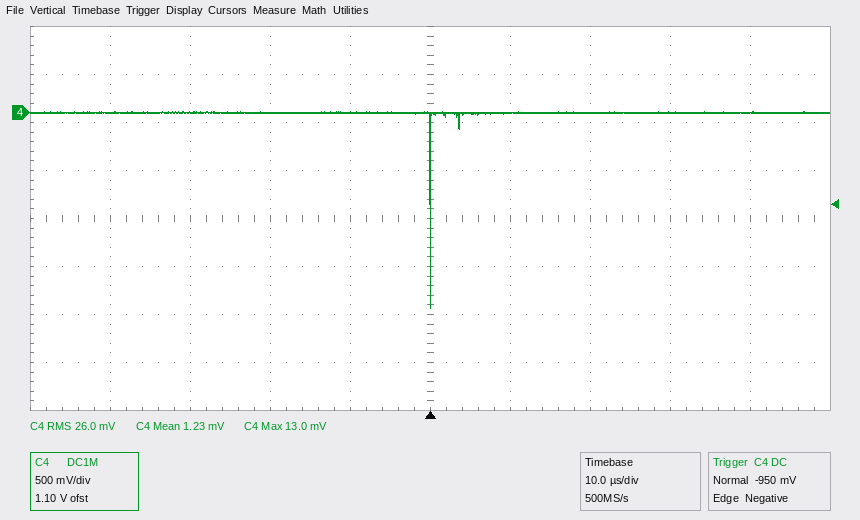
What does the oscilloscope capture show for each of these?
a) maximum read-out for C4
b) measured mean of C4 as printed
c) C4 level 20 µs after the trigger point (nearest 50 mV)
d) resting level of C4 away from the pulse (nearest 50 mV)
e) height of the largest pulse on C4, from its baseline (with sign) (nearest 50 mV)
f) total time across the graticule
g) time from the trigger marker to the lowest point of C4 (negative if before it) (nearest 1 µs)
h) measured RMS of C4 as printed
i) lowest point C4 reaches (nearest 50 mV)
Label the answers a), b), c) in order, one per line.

a) 13.0 mV
b) 1.23 mV
c) 0 mV
d) 0 mV
e) -2.05 V
f) 100 µs
g) 0 µs
h) 26.0 mV
i) -2.05 V
